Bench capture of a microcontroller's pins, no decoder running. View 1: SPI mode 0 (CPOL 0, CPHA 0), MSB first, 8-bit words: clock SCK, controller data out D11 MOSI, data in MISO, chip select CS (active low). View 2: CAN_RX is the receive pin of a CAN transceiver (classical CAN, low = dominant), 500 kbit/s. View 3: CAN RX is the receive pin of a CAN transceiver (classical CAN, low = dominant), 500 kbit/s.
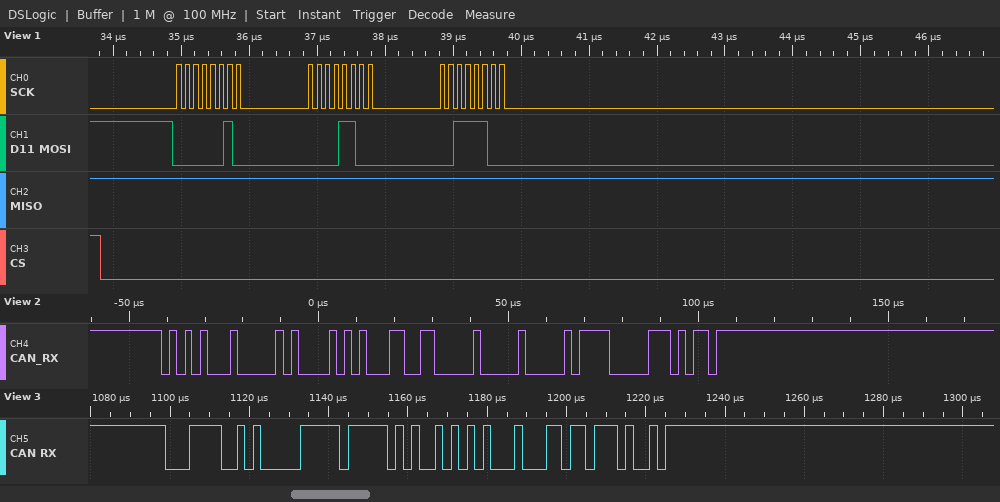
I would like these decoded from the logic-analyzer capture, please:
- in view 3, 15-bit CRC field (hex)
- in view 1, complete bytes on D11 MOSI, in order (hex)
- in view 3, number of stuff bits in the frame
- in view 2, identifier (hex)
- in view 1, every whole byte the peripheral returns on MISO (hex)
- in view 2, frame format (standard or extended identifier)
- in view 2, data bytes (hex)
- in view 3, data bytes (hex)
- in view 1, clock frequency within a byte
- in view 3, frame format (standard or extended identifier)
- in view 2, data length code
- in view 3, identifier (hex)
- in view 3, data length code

0x1B74
02 0C 3C
3
0x544
FF FF FF
standard
2A 33 00 00
FF 4A A2
8 MHz
standard
4
0x1E5
3
